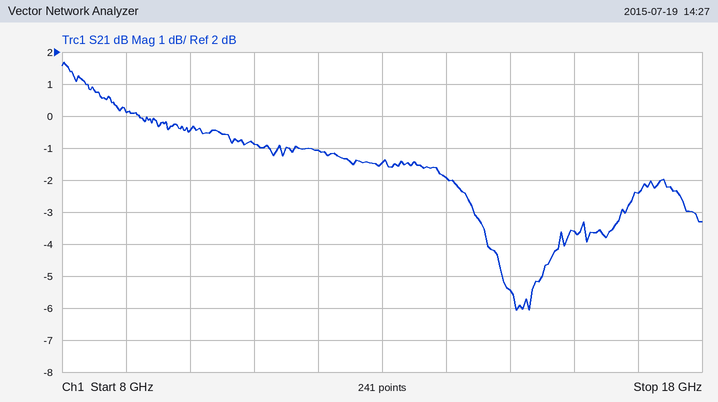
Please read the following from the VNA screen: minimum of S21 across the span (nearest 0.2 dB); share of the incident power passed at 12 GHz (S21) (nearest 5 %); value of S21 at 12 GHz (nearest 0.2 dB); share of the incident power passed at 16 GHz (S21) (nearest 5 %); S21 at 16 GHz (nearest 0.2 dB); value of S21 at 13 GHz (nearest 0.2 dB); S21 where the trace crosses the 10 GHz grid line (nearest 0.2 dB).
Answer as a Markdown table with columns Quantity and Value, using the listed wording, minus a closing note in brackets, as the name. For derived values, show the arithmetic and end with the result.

| Quantity | Value |
|---|---|
| minimum of S21 across the span | -6.0 dB |
| share of the incident power passed at 12 GHz (S21) | 10^(-1/10) ≈ 79.4 %, so 80 % to the nearest 5 % |
| value of S21 at 12 GHz | -1.0 dB |
| share of the incident power passed at 16 GHz (S21) | 10^(-3.6/10) ≈ 43.7 %, so 45 % to the nearest 5 % |
| S21 at 16 GHz | -3.6 dB |
| value of S21 at 13 GHz | -1.4 dB |
| S21 where the trace crosses the 10 GHz grid line | -0.4 dB |
